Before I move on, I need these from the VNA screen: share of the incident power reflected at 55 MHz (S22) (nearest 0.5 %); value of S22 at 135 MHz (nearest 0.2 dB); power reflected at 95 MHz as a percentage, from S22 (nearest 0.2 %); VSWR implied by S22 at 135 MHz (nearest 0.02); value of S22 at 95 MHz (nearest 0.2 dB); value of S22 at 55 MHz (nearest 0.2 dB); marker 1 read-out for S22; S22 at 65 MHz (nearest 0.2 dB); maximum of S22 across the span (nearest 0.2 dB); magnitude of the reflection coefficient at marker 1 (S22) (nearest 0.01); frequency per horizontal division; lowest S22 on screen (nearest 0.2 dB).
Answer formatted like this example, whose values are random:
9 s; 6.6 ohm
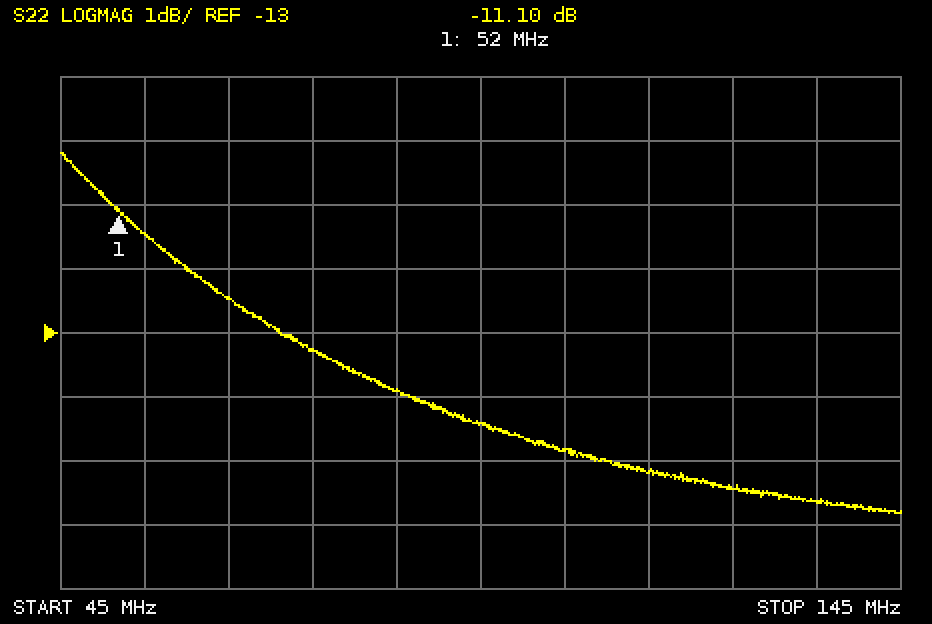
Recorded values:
7.0 %; -15.6 dB; 3.6 %; 1.40; -14.4 dB; -11.4 dB; -11.10 dB; -12.4 dB; -10.2 dB; 0.28; 10 MHz; -15.8 dB
